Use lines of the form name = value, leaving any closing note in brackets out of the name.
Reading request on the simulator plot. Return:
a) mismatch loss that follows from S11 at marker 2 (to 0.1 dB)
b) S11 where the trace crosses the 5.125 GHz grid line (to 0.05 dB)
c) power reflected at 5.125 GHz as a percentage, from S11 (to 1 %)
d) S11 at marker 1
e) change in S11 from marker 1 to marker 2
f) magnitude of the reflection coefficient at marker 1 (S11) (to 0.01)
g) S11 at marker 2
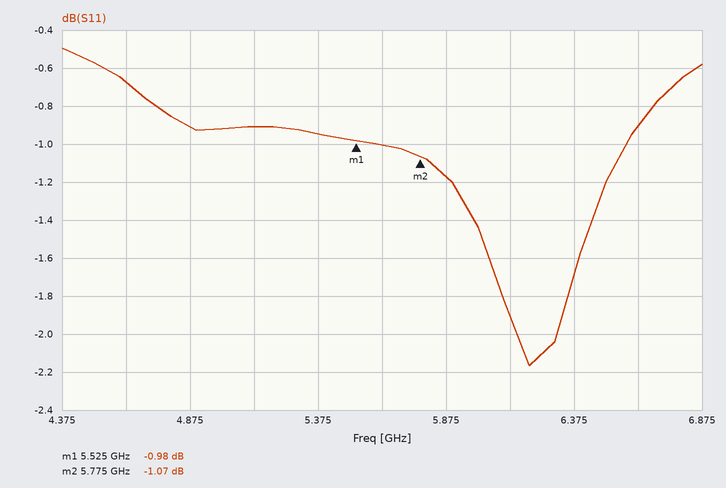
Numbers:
mismatch loss that follows from S11 at marker 2 = 6.6 dB
S11 where the trace crosses the 5.125 GHz grid line = -0.90 dB
power reflected at 5.125 GHz as a percentage, from S11 = 81 %
S11 at marker 1 = -0.98 dB
change in S11 from marker 1 to marker 2 = -0.09 dB
magnitude of the reflection coefficient at marker 1 (S11) = 0.89
S11 at marker 2 = -1.07 dB
